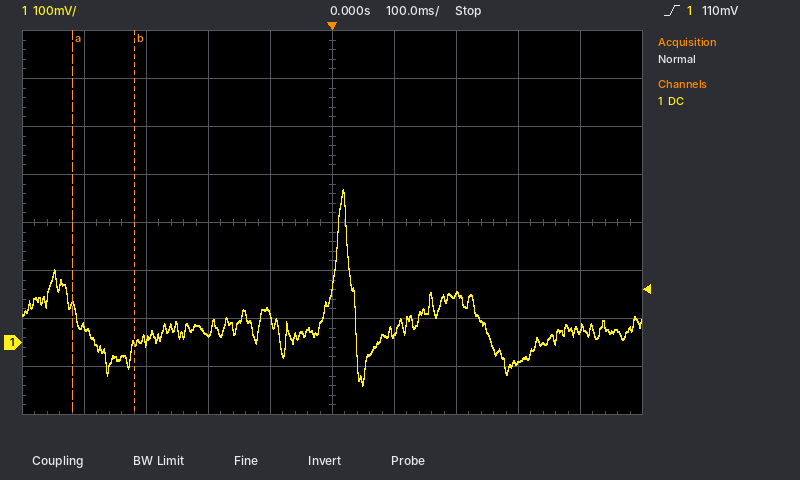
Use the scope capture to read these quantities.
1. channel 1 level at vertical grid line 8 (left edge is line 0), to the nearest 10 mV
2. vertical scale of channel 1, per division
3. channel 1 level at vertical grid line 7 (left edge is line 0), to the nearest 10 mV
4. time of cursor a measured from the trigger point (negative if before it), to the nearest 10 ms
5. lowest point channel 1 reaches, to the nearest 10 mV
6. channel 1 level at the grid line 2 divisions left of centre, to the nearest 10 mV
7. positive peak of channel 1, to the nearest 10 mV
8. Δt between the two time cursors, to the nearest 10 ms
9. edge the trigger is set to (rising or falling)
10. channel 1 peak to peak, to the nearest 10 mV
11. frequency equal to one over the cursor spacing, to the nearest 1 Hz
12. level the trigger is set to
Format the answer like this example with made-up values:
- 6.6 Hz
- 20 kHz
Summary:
- -40 mV
- 100 mV
- 100 mV
- -420 ms
- -90 mV
- 20 mV
- 320 mV
- 100 ms
- rising
- 410 mV
- 10 Hz
- 110 mV
